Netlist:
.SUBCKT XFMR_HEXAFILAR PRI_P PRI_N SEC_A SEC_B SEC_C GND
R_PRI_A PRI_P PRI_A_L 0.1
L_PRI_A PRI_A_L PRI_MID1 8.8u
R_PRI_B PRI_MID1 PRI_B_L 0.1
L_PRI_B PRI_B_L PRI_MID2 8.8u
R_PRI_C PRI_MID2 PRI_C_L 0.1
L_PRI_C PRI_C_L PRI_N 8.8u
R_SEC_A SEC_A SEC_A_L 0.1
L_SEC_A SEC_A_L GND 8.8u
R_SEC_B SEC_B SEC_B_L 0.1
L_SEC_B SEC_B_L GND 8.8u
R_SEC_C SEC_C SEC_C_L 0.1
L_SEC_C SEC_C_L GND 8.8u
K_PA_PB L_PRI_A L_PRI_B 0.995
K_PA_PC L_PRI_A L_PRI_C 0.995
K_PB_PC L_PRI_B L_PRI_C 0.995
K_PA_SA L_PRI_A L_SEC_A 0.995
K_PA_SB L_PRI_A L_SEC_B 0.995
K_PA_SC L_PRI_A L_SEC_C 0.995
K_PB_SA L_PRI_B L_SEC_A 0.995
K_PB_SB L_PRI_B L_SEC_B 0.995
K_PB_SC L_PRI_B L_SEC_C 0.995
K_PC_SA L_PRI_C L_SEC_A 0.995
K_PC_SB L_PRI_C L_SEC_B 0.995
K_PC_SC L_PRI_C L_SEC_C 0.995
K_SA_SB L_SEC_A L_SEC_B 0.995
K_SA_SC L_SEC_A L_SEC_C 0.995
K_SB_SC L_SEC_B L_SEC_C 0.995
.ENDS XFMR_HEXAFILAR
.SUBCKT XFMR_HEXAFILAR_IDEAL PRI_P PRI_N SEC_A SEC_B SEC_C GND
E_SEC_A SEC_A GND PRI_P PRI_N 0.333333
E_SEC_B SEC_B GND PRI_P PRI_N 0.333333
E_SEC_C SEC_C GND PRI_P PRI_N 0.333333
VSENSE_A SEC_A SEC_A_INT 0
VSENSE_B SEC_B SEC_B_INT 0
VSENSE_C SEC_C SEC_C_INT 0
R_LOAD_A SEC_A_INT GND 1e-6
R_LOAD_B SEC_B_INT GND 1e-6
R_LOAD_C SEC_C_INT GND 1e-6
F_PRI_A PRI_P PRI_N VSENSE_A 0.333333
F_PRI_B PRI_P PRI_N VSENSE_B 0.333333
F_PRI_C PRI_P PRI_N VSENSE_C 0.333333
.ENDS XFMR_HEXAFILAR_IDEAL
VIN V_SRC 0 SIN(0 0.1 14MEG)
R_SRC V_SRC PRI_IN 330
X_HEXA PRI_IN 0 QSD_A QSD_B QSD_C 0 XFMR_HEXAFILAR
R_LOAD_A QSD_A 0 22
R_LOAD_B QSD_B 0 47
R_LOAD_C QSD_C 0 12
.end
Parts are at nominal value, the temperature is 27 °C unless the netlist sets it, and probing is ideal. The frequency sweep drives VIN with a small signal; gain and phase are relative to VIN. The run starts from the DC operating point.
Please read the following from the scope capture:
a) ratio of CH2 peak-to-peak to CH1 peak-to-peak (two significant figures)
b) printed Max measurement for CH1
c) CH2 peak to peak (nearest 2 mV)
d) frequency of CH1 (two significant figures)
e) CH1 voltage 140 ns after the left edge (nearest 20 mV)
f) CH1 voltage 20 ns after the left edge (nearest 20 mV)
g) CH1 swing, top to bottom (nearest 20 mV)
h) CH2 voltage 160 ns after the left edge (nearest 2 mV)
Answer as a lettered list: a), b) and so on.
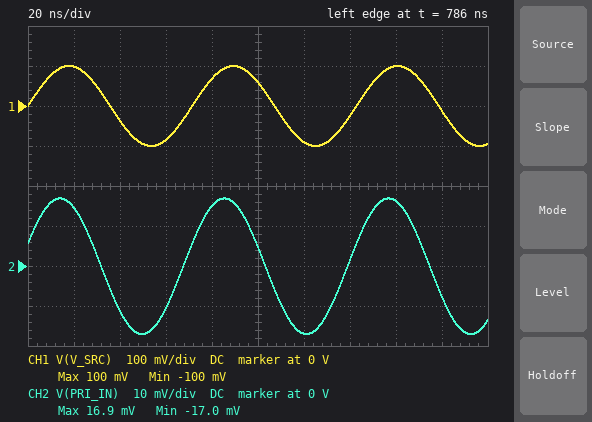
a) 0.17
b) 100 mV
c) 34 mV
d) 14 MHz
e) -20 mV
f) 100 mV
g) 200 mV
h) 16 mV
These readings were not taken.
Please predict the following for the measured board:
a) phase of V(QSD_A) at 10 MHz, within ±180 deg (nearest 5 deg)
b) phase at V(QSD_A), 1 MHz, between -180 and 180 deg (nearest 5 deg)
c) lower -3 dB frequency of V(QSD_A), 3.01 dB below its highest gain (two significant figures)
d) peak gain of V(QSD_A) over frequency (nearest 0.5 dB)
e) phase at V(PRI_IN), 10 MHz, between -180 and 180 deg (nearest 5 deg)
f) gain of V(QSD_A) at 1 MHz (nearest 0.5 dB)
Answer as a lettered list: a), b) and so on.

a) 0 deg
b) 5 deg
c) 130 kHz
d) -25.0 dB
e) 15 deg
f) -26.0 dB
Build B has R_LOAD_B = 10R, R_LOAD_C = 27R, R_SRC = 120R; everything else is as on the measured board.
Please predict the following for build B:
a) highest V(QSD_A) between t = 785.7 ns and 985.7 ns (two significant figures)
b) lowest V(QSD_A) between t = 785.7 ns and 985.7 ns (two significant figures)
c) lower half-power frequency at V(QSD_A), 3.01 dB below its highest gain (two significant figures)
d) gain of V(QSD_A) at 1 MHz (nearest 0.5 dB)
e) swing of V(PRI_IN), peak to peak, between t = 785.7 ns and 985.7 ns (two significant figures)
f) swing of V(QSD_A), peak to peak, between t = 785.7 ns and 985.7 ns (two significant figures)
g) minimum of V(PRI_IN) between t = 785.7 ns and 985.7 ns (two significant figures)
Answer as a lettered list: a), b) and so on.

a) 9.8 mV
b) -9.9 mV
c) 81 kHz
d) -20.5 dB
e) 66 mV
f) 20 mV
g) -33 mV
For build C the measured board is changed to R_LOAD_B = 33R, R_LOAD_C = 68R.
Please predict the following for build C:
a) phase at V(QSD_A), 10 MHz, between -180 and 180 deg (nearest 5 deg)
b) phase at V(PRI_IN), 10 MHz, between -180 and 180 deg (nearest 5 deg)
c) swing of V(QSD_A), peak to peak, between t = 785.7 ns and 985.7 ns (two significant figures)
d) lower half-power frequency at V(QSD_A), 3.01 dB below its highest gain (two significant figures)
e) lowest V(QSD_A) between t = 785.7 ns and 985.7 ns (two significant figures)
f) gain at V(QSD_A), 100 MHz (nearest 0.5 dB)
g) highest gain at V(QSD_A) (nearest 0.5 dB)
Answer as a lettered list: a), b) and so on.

a) -5 deg
b) 10 deg
c) 15 mV
d) 150 kHz
e) -7.7 mV
f) -24.0 dB
g) -22.5 dB
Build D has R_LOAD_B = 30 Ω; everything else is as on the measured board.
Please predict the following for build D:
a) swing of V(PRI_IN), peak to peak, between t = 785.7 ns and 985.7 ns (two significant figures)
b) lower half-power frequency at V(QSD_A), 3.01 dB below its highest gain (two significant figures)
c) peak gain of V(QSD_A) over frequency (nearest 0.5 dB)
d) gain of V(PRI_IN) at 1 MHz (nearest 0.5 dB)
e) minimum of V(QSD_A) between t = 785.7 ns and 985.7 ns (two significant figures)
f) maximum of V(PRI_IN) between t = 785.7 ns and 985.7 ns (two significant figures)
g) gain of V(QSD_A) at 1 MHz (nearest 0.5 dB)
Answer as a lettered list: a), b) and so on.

a) 32 mV
b) 120 kHz
c) -25.5 dB
d) -17.0 dB
e) -4.9 mV
f) 16 mV
g) -26.5 dB
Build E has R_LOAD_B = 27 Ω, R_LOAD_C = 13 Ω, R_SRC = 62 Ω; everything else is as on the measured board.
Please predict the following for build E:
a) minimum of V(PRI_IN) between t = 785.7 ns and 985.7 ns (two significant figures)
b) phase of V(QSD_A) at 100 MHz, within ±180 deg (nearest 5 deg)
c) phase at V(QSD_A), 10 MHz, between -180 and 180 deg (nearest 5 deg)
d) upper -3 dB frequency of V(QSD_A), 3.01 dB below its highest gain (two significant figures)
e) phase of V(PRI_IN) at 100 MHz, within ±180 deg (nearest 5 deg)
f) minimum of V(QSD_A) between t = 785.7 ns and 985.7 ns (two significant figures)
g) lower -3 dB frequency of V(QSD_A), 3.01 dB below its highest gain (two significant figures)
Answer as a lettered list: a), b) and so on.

a) -51 mV
b) -50 deg
c) -5 deg
d) 88 MHz
e) 15 deg
f) -16 mV
g) 60 kHz
